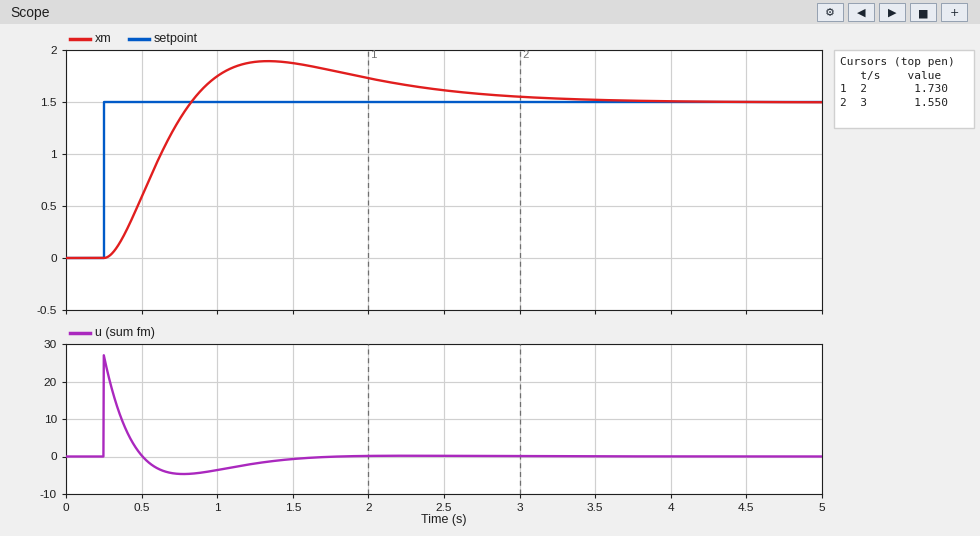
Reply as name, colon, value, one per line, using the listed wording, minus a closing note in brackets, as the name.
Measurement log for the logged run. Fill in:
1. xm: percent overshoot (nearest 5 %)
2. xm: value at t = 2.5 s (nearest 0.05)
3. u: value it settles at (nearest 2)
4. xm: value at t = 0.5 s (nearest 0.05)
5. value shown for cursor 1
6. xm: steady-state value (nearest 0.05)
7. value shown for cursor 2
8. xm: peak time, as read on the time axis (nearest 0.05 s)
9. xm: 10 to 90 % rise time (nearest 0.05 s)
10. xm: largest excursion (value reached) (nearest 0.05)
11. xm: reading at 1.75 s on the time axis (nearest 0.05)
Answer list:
xm: percent overshoot: 25 %
xm: value at t = 2.5 s: 1.60
u: value it settles at: 0
xm: value at t = 0.5 s: 0.60
value shown for cursor 1: 1.730
xm: steady-state value: 1.50
value shown for cursor 2: 1.550
xm: peak time, as read on the time axis: 1.35 s
xm: 10 to 90 % rise time: 0.40 s
xm: largest excursion (value reached): 1.90
xm: reading at 1.75 s on the time axis: 1.80
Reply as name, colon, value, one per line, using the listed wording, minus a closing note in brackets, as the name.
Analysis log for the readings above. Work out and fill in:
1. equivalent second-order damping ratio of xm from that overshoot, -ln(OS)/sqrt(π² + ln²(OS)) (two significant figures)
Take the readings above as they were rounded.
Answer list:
equivalent second-order damping ratio of xm from that overshoot, -ln(OS)/sqrt(π² + ln²(OS)): 0.40
